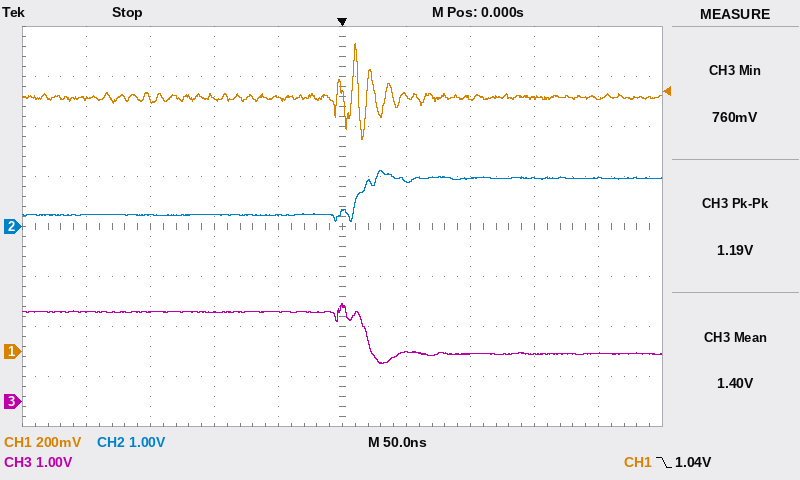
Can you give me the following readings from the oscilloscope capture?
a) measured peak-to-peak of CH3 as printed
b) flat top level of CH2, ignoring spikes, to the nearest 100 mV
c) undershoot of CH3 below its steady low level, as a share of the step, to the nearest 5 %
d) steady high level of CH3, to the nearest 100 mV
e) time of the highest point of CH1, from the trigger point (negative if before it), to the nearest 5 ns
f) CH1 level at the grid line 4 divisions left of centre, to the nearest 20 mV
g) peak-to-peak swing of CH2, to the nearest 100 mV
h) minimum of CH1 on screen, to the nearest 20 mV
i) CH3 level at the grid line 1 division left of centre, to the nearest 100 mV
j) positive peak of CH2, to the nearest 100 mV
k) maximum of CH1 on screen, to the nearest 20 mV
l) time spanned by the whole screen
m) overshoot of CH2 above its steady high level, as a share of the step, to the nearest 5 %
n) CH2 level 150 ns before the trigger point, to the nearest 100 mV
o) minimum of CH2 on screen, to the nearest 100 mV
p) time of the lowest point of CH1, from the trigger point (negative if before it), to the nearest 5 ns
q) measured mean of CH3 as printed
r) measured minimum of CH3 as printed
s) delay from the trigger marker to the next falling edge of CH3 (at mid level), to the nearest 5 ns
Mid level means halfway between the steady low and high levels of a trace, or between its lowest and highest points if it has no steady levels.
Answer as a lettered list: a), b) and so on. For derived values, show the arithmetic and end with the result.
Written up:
a) 1.19 V
b) 1.0 V
c) 25 %
d) 1.8 V
e) +10 ns
f) 1.02 V
g) 1.1 V − (100 mV) = 1.0 V
h) 840 mV
i) 1.8 V
j) 1.1 V
k) 1.24 V
l) 500 ns
m) 20 %
n) 200 mV
o) 100 mV
p) +15 ns
q) 1.40 V
r) 760 mV
s) 20 ns
